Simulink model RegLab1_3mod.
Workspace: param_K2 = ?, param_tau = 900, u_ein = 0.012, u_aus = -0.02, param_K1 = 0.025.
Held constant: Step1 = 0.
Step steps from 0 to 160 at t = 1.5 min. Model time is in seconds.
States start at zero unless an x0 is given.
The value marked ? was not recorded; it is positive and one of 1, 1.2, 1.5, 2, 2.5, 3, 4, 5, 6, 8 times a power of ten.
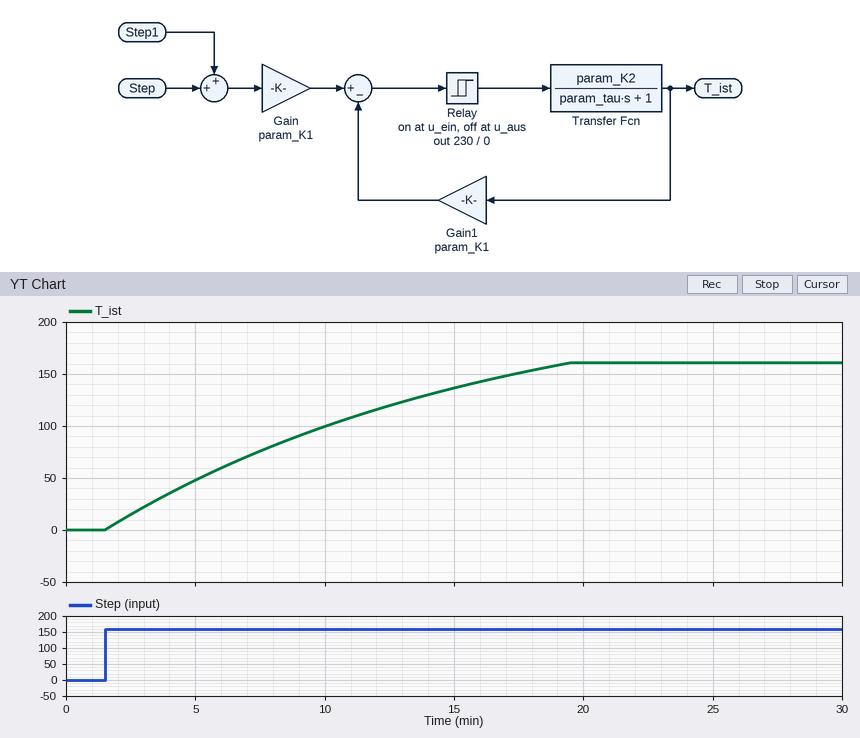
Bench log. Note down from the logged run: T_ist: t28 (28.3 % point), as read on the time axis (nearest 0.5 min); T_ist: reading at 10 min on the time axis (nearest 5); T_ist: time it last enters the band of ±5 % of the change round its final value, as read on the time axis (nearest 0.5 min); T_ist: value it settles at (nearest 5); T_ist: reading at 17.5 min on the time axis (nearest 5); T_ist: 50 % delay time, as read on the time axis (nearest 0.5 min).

5.0 min
100
18.0 min
160
150
8.0 min
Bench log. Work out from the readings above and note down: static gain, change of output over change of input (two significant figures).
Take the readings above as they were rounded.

1.0
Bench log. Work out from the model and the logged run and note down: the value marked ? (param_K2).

1
